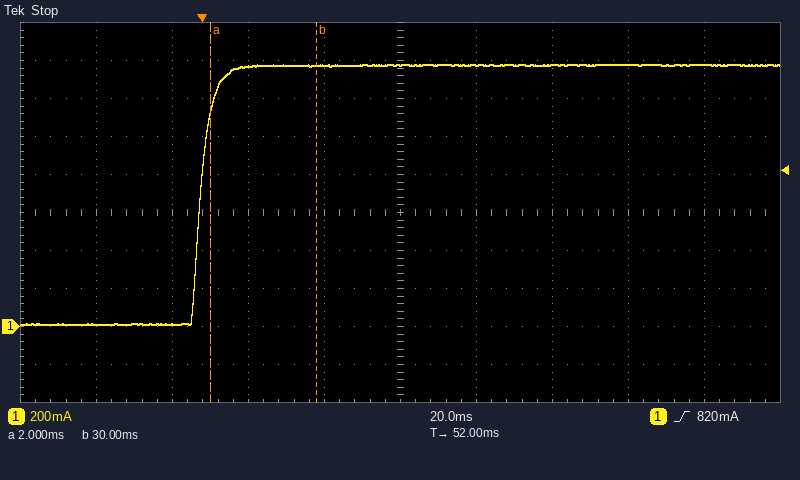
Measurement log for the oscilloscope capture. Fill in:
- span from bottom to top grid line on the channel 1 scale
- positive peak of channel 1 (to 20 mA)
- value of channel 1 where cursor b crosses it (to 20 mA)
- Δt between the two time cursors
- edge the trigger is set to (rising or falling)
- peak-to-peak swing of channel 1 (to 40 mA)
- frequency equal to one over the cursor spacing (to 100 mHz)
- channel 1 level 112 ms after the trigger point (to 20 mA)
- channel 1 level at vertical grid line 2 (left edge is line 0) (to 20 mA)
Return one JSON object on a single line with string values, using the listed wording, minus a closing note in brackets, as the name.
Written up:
{"span from bottom to top grid line on the channel 1 scale": "2 A", "positive peak of channel 1": "1.38 A", "value of channel 1 where cursor b crosses it": "1.38 A", "Δt between the two time cursors": "28 ms", "edge the trigger is set to": "rising", "peak-to-peak swing of channel 1": "1.36 A", "frequency equal to one over the cursor spacing": "35.7 Hz", "channel 1 level 112 ms after the trigger point": "1.38 A", "channel 1 level at vertical grid line 2 (left edge is line 0)": "20 mA"}
